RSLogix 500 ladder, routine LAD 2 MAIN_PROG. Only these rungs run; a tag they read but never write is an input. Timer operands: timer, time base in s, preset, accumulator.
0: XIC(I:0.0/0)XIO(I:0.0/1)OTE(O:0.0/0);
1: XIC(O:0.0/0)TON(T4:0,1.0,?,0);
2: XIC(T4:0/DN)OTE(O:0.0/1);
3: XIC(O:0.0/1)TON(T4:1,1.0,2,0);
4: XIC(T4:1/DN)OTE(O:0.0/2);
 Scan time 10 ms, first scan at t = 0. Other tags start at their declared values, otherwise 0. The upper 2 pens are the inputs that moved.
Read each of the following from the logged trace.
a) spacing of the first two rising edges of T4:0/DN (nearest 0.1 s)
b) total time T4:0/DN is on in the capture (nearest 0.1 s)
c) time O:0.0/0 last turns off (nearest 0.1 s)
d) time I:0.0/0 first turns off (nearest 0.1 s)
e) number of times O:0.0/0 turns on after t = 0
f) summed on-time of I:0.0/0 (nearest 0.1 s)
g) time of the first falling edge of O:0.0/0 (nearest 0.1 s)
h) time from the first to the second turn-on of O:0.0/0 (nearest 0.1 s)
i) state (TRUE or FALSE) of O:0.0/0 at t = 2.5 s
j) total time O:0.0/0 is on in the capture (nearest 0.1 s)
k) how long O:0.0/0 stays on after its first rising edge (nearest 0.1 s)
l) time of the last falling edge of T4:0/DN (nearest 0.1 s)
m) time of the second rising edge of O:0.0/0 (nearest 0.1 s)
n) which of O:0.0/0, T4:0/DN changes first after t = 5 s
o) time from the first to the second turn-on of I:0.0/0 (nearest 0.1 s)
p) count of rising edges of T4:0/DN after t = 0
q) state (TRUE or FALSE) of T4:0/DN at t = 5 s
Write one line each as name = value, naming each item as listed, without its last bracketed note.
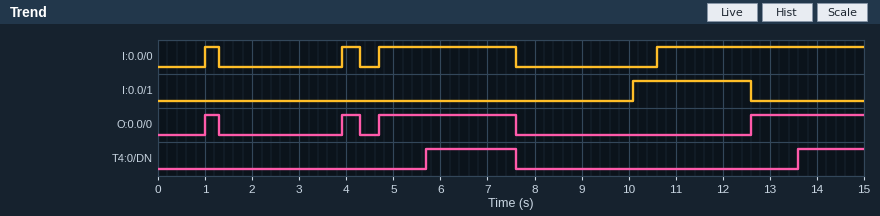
spacing of the first two rising edges of T4:0/DN = 7.9 s
total time T4:0/DN is on in the capture = 3.3 s
time O:0.0/0 last turns off = 7.6 s
time I:0.0/0 first turns off = 1.3 s
number of times O:0.0/0 turns on after t = 0 = 4
summed on-time of I:0.0/0 = 8.0 s
time of the first falling edge of O:0.0/0 = 1.3 s
time from the first to the second turn-on of O:0.0/0 = 2.9 s
state (TRUE or FALSE) of O:0.0/0 at t = 2.5 s = FALSE
total time O:0.0/0 is on in the capture = 6.0 s
how long O:0.0/0 stays on after its first rising edge = 0.3 s
time of the last falling edge of T4:0/DN = 7.6 s
time of the second rising edge of O:0.0/0 = 3.9 s
which of O:0.0/0, T4:0/DN changes first after t = 5 s = T4:0/DN
time from the first to the second turn-on of I:0.0/0 = 2.9 s
count of rising edges of T4:0/DN after t = 0 = 2
state (TRUE or FALSE) of T4:0/DN at t = 5 s = FALSE
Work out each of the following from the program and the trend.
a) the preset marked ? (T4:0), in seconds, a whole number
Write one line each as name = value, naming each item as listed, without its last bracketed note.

the preset marked ? (T4:0), in seconds, a whole number = 1 s
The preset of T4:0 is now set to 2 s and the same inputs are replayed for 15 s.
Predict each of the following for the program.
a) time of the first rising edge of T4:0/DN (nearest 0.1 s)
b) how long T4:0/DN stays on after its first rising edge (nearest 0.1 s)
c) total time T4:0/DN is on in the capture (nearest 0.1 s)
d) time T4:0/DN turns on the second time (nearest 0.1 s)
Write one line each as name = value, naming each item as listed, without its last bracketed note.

time of the first rising edge of T4:0/DN = 6.7 s
how long T4:0/DN stays on after its first rising edge = 0.9 s
total time T4:0/DN is on in the capture = 1.3 s
time T4:0/DN turns on the second time = 14.6 s
